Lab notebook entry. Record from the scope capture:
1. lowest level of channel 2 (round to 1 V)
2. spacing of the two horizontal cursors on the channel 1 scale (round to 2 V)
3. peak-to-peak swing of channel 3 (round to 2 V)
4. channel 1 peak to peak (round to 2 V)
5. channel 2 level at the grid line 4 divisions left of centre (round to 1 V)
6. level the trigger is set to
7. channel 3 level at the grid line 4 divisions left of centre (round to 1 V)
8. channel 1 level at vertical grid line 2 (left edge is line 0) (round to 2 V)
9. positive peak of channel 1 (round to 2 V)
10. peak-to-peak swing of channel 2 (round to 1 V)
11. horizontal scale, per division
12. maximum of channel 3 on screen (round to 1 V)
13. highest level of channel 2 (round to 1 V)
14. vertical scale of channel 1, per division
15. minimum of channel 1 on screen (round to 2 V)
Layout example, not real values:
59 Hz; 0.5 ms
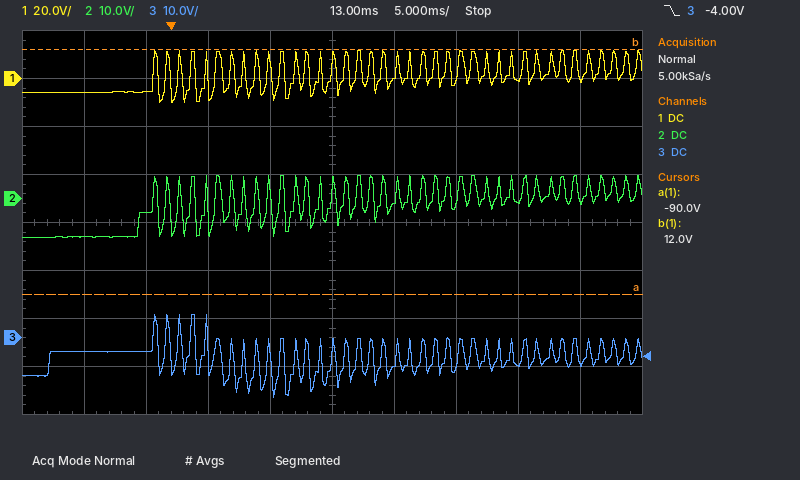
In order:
-8 V; 102 V; 18 V; 22 V; -8 V; -4.00 V; -3 V; -6 V; 12 V; 13 V; 5 ms; 5 V; 5 V; 20 V; -10 V
